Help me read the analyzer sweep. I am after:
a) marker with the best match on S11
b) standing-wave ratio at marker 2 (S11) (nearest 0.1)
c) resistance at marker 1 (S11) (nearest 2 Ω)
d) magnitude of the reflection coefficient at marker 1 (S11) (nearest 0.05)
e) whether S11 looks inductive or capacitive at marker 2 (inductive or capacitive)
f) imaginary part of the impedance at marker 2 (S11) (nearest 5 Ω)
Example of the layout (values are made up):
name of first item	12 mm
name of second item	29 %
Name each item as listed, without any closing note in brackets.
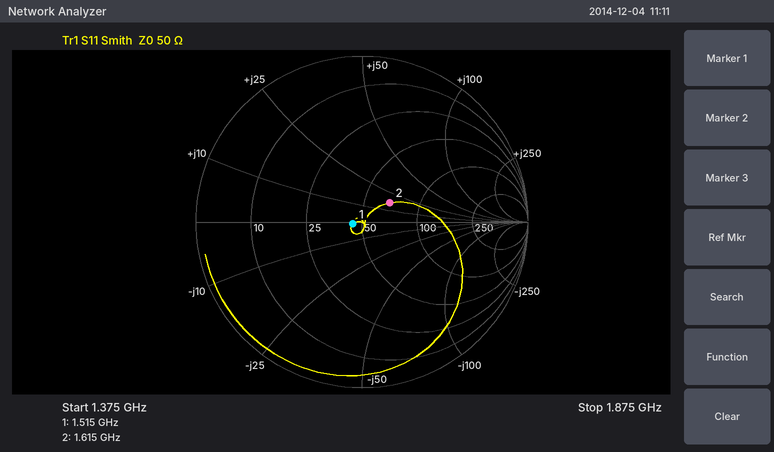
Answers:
marker with the best match on S11	marker 1
standing-wave ratio at marker 2 (S11)	1.5
resistance at marker 1 (S11)	44 Ω
magnitude of the reflection coefficient at marker 1 (S11)	0.05
whether S11 looks inductive or capacitive at marker 2	inductive
imaginary part of the impedance at marker 2 (S11)	+15 Ω
